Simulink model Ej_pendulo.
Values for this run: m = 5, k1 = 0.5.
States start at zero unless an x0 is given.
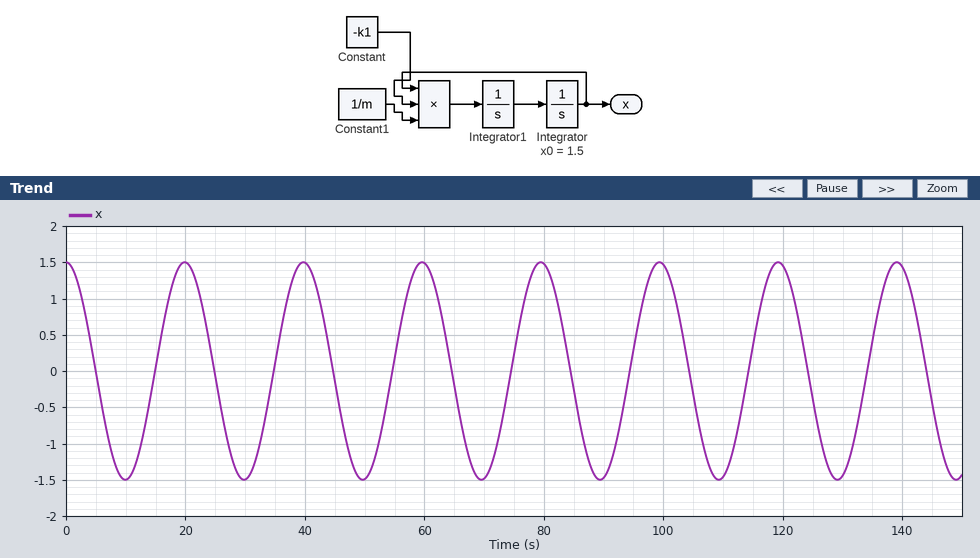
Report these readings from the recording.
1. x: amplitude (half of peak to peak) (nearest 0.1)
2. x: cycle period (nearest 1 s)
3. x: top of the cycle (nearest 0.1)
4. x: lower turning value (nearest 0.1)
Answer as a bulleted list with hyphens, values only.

- 1.5
- 20 s
- 1.5
- -1.5
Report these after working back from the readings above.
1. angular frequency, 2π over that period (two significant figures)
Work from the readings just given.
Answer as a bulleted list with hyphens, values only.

- 0.31 rad/s
